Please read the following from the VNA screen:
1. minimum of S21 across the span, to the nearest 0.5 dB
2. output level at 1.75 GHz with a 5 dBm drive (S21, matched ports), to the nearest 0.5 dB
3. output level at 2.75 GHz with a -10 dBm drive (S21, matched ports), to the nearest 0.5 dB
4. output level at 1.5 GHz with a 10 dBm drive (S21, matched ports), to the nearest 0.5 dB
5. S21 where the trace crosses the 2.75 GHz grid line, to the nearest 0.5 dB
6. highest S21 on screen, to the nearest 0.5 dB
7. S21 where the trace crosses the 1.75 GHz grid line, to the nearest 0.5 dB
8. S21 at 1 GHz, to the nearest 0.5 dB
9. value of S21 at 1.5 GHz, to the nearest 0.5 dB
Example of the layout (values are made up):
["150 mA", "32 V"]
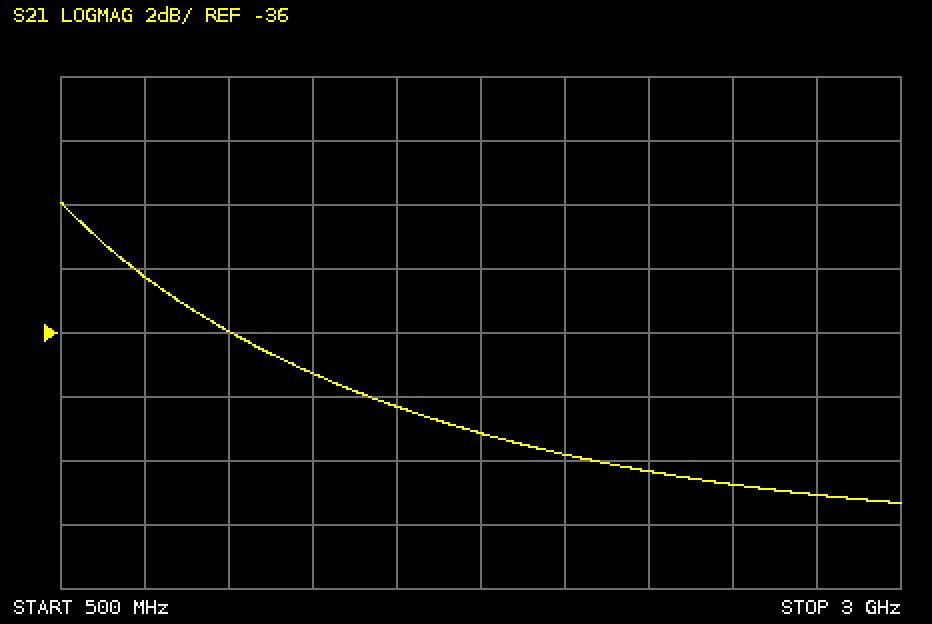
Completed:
["-41.5 dB", "-34.0 dBm", "-51.0 dBm", "-28.5 dBm", "-41.0 dB", "-32.0 dB", "-39.0 dB", "-36.0 dB", "-38.5 dB"]
